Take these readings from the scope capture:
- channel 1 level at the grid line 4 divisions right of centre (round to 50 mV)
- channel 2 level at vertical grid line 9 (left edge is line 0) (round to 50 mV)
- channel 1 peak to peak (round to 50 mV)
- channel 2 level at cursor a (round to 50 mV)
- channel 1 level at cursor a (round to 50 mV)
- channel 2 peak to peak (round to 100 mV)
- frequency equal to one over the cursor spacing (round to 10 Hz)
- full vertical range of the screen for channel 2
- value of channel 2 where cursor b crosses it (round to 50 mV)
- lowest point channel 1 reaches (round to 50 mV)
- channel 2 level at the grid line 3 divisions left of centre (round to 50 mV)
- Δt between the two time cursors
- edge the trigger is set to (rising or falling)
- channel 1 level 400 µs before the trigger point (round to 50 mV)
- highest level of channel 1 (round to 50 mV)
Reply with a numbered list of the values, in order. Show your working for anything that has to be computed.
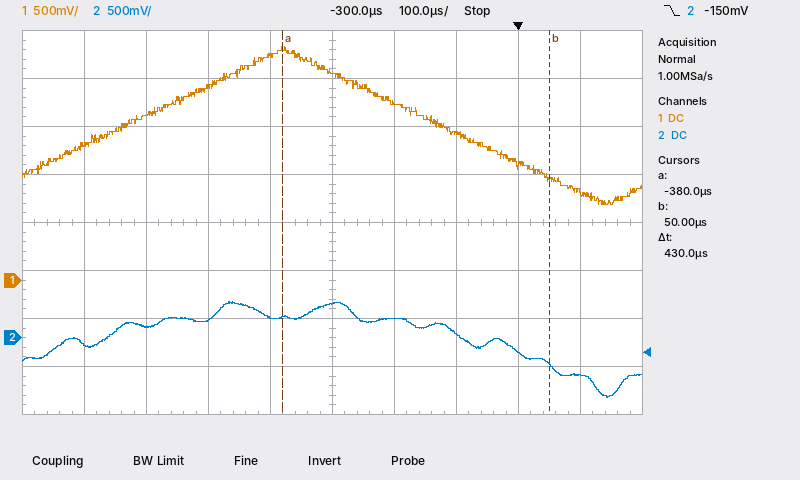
1. 900 mV
2. -400 mV
3. 2.45 V − (800 mV) = 1.65 V
4. 200 mV
5. 2.40 V
6. 1.00 V
7. 1 / 430 µs ≈ 2.33 kHz
8. 4 V
9. -300 mV
10. 800 mV
11. 100 mV
12. 430 µs
13. falling
14. 2.35 V
15. 2.45 V
